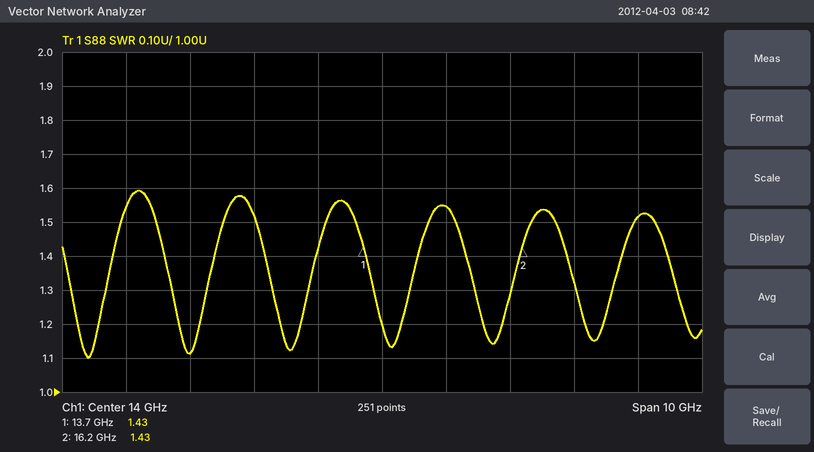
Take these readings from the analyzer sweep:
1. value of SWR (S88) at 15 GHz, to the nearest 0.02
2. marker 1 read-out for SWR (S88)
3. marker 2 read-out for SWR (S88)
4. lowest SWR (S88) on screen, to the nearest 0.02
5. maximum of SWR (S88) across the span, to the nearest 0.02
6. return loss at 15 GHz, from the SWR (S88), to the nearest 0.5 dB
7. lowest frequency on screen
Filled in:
1.54
1.43
1.43
1.10
1.60
13.5 dB
9 GHz
